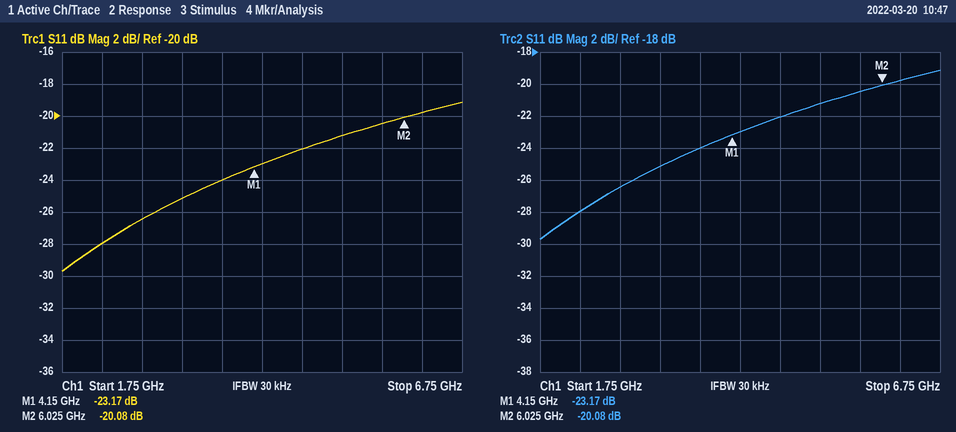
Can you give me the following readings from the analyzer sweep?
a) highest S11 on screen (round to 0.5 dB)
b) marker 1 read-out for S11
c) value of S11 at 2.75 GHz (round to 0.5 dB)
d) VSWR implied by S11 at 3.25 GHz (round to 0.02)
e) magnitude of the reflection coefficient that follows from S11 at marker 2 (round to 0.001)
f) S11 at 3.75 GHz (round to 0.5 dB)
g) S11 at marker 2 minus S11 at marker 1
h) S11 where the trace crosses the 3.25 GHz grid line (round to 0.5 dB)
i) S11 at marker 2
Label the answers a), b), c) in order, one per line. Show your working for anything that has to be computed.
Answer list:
a) -19.0 dB
b) -23.17 dB
c) -26.5 dB
d) |Γ| = 10^(-25/20) = 0.0562; VSWR = (1 + 0.0562)/(1 − 0.0562) ≈ 1.12
e) 10^(-20.08/20) ≈ 0.099
f) -24.0 dB
g) -20.08 − (-23.17) = 3.09 dB
h) -25.0 dB
i) -20.08 dB
